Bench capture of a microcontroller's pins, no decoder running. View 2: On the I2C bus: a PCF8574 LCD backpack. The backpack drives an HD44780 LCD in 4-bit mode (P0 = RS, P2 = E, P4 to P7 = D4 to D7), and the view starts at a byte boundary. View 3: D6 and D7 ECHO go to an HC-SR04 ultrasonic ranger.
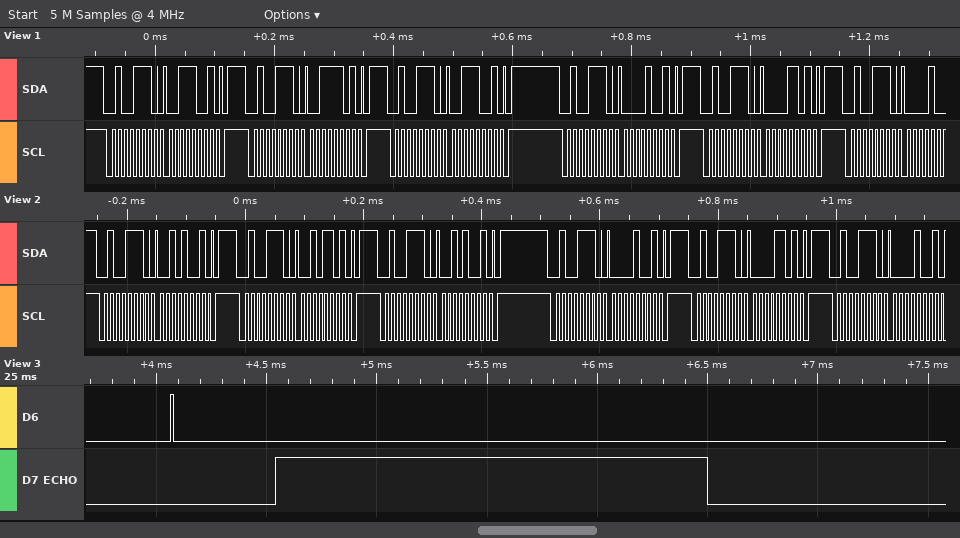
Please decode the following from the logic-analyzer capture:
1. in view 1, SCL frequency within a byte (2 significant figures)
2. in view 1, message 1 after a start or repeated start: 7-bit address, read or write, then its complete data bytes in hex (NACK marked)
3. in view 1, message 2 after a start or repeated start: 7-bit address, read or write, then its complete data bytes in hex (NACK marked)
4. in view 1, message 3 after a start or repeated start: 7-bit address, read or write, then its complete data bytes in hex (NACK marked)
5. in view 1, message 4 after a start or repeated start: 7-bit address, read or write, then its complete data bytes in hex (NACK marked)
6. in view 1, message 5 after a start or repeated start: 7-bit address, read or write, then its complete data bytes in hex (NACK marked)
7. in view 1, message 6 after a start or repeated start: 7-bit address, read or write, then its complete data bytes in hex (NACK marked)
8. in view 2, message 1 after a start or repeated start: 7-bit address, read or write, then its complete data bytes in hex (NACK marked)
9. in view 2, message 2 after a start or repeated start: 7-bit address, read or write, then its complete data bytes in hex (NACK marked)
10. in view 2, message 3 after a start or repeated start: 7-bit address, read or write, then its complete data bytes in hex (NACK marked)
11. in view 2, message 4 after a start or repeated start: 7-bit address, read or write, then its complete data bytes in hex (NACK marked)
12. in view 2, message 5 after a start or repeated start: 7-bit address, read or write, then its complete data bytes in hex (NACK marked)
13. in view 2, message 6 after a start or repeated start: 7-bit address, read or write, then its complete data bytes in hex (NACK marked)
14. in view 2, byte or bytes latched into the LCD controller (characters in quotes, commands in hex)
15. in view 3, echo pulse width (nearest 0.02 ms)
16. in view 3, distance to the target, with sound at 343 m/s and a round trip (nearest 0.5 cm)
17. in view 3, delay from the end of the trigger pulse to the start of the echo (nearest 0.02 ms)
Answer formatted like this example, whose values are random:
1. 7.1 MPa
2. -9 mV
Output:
1. 100 kHz
2. 0x27 write: 39
3. 0x27 write: 3D
4. 0x27 write: 39
5. 0x27 write: 09
6. 0x27 write: 0D
7. 0x27 write
8. 0x27 write: 29
9. 0x27 write: 2D
10. 0x27 write: 29
11. 0x27 write: 09
12. 0x27 write: 0D
13. 0x27 write: 09
14. ' '
15. 1.96 ms
16. 33.5 cm
17. 0.46 ms
